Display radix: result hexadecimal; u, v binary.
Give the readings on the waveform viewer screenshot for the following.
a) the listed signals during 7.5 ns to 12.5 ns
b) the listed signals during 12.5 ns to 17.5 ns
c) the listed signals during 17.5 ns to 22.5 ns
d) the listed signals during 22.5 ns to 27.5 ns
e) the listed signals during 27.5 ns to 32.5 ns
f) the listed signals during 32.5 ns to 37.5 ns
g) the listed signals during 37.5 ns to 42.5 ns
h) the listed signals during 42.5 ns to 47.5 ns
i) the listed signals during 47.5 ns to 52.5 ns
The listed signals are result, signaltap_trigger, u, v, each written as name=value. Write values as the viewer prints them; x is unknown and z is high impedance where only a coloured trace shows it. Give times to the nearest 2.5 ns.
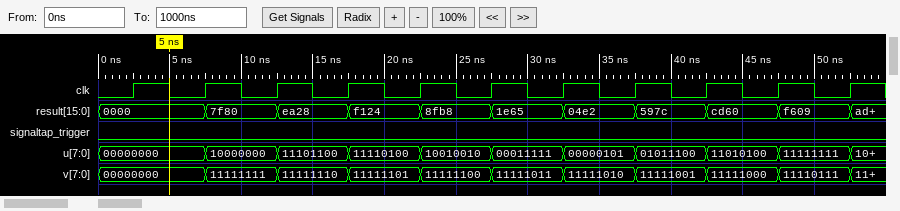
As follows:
result=7f80, signaltap_trigger=0, u=10000000, v=11111111
result=ea28, signaltap_trigger=0, u=11101100, v=11111110
result=f124, signaltap_trigger=0, u=11110100, v=11111101
result=8fb8, signaltap_trigger=0, u=10010010, v=11111100
result=1e65, signaltap_trigger=0, u=00011111, v=11111011
result=04e2, signaltap_trigger=0, u=00000101, v=11111010
result=597c, signaltap_trigger=0, u=01011100, v=11111001
result=cd60, signaltap_trigger=0, u=11010100, v=11111000
result=f609, signaltap_trigger=0, u=11111111, v=11110111
